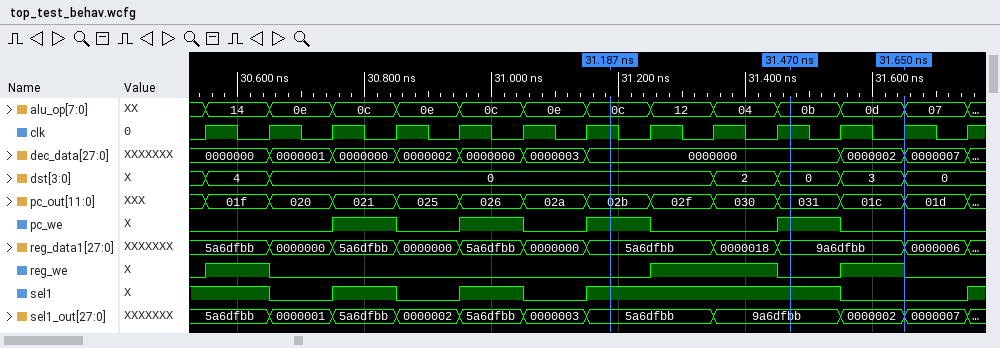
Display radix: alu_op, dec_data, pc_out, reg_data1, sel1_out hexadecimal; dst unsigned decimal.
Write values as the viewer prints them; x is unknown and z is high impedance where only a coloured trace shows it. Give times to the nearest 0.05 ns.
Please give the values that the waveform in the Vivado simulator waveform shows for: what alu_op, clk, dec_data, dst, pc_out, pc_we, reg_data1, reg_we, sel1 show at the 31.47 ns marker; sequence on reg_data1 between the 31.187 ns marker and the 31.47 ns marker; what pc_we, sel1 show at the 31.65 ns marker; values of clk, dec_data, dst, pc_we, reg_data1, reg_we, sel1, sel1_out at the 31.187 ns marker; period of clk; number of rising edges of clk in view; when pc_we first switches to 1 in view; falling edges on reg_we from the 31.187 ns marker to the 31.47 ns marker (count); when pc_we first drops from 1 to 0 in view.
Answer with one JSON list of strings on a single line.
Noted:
["alu_op=0b, clk=1, dec_data=0000000, dst=0, pc_out=031, pc_we=1, reg_data1=9a6dfbb, reg_we=0, sel1=1", "5a6dfbb, 0000018, 9a6dfbb", "pc_we=0, sel1=0", "clk=1, dec_data=0000000, dst=0, pc_we=1, reg_data1=5a6dfbb, reg_we=0, sel1=1, sel1_out=5a6dfbb", "0.1 ns", "13", "30.75 ns", "1", "30.85 ns"]
